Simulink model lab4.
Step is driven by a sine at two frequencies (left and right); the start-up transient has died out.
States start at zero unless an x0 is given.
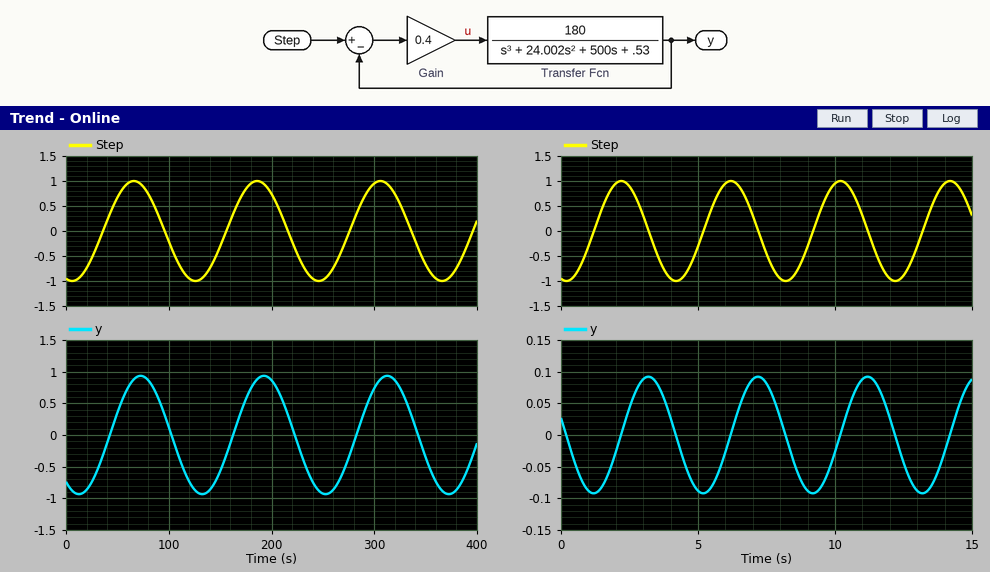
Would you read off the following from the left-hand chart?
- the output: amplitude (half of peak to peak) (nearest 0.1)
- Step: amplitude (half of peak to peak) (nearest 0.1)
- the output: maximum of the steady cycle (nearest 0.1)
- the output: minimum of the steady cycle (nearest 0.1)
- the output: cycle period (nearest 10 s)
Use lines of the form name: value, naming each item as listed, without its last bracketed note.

the output: amplitude (half of peak to peak): 0.9
Step: amplitude (half of peak to peak): 1.0
the output: maximum of the steady cycle: 0.9
the output: minimum of the steady cycle: -0.9
the output: cycle period: 120 s
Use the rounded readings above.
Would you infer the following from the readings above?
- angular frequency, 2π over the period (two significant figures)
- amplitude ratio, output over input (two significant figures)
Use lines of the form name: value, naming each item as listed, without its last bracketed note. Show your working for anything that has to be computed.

angular frequency, 2π over the period: 2π / 120 = 0.052 rad/s
amplitude ratio, output over input: 0.9 / 1 = 0.90
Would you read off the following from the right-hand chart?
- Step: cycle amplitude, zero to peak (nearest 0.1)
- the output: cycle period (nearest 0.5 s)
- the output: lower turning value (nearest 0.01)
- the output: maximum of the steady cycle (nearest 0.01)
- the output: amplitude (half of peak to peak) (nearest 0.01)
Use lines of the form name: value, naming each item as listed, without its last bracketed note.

Step: cycle amplitude, zero to peak: 1.0
the output: cycle period: 4.0 s
the output: lower turning value: -0.09
the output: maximum of the steady cycle: 0.09
the output: amplitude (half of peak to peak): 0.09
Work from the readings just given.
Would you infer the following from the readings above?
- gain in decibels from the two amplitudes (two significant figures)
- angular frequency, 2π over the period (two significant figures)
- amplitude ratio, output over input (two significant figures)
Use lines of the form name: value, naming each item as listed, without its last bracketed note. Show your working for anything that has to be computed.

gain in decibels from the two amplitudes: 20 log10(0.09 / 1) = -21 dB
angular frequency, 2π over the period: 2π / 4 = 1.6 rad/s
amplitude ratio, output over input: 0.09 / 1 = 0.090
